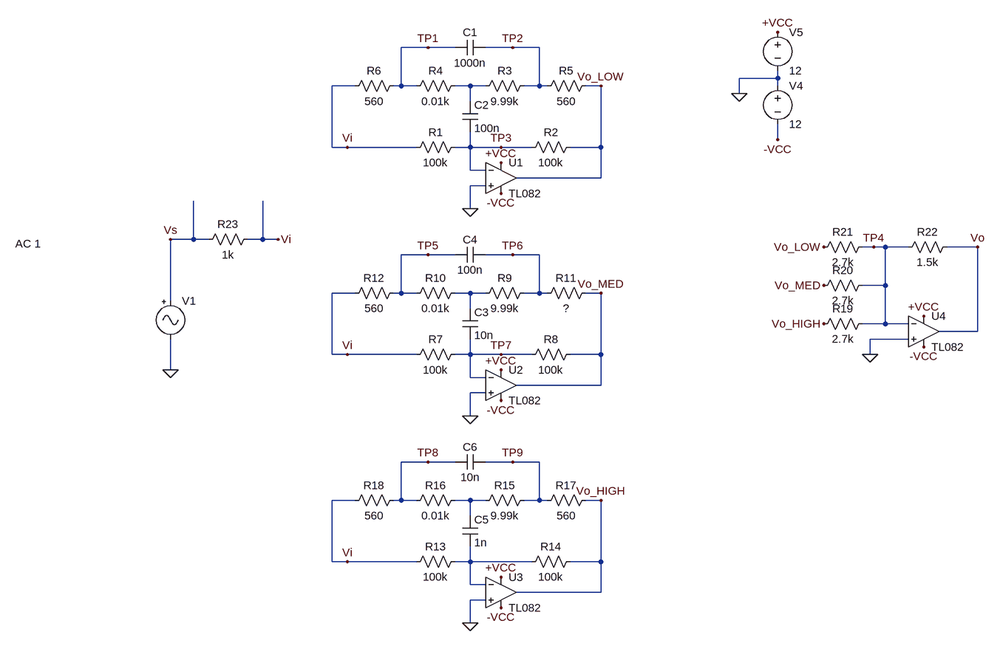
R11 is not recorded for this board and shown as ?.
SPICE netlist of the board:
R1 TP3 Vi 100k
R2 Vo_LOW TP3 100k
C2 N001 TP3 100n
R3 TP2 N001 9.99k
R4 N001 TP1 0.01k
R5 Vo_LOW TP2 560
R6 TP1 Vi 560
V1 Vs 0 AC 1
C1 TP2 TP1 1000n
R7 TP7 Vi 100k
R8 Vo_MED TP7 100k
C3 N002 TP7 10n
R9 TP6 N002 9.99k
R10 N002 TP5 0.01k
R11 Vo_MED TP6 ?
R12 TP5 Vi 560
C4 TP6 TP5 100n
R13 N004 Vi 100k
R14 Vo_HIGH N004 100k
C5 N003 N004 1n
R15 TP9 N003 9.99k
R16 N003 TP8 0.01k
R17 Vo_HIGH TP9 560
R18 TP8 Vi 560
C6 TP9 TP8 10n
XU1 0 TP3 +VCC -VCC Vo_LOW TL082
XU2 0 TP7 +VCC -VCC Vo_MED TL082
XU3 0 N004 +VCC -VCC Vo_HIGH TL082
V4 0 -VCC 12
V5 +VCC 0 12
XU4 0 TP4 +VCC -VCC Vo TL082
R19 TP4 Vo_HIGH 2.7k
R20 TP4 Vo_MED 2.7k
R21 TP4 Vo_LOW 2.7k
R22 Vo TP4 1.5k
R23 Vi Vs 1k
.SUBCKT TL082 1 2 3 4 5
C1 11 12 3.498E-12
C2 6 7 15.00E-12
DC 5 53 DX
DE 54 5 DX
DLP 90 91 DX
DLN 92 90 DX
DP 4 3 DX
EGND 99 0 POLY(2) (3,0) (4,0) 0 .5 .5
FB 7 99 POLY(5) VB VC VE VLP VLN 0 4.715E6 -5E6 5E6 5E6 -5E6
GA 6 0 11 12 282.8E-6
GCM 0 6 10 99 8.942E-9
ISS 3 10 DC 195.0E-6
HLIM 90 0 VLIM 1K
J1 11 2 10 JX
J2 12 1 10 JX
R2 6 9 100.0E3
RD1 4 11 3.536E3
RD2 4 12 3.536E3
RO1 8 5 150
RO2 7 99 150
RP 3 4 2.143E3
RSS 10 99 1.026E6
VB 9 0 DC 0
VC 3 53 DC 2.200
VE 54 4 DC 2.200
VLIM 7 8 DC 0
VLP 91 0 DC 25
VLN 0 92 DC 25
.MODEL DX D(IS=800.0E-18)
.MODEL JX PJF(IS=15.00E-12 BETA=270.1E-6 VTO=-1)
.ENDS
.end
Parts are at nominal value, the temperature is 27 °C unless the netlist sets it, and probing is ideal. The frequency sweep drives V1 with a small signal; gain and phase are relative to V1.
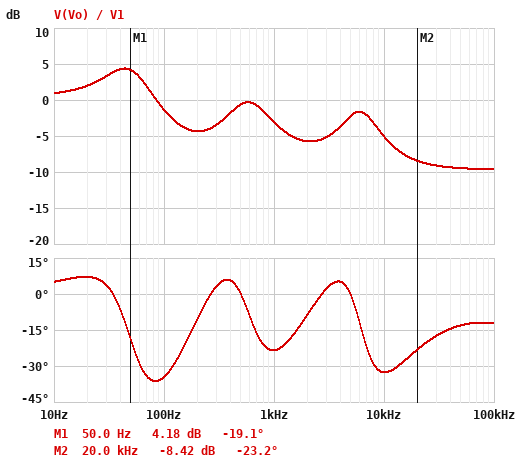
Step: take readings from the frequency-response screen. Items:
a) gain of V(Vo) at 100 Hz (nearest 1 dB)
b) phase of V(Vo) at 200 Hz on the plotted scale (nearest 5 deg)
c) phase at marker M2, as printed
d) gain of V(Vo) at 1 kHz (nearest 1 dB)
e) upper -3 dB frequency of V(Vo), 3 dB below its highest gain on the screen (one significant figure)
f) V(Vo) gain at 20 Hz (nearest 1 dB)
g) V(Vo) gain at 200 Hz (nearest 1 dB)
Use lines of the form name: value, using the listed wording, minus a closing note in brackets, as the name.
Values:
gain of V(Vo) at 100 Hz: -1 dB
phase of V(Vo) at 200 Hz on the plotted scale: -10 deg
phase at marker M2, as printed: -23.2 deg
gain of V(Vo) at 1 kHz: -3 dB
upper -3 dB frequency of V(Vo), 3 dB below its highest gain on the screen: 70 Hz
V(Vo) gain at 20 Hz: 2 dB
V(Vo) gain at 200 Hz: -4 dB
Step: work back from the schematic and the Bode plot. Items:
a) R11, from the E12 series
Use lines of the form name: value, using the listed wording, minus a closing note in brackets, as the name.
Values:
R11, from the E12 series: 1 kΩ
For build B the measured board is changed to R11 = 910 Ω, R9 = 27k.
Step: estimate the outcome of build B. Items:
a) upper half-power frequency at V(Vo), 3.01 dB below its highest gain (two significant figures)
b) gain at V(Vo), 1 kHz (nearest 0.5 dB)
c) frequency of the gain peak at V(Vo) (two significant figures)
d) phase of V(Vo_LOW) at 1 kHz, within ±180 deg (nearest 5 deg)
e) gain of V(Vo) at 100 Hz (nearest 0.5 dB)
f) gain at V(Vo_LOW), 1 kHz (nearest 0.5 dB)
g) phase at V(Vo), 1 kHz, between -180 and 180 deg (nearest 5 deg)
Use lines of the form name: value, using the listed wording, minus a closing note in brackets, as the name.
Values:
upper half-power frequency at V(Vo), 3.01 dB below its highest gain: 72 Hz
gain at V(Vo), 1 kHz: -3.5 dB
frequency of the gain peak at V(Vo): 43 Hz
phase of V(Vo_LOW) at 1 kHz, within ±180 deg: 155 deg
gain of V(Vo) at 100 Hz: -1.0 dB
gain at V(Vo_LOW), 1 kHz: -14.5 dB
phase at V(Vo), 1 kHz, between -180 and 180 deg: -30 deg
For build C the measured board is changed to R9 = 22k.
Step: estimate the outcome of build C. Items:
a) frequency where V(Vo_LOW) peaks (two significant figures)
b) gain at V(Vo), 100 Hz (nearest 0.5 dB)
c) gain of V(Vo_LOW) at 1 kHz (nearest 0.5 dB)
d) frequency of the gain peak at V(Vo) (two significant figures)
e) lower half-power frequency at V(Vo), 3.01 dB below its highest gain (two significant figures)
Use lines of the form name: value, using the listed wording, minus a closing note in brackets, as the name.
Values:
frequency where V(Vo_LOW) peaks: 48 Hz
gain at V(Vo), 100 Hz: -1.0 dB
gain of V(Vo_LOW) at 1 kHz: -14.5 dB
frequency of the gain peak at V(Vo): 43 Hz
lower half-power frequency at V(Vo), 3.01 dB below its highest gain: 13 Hz
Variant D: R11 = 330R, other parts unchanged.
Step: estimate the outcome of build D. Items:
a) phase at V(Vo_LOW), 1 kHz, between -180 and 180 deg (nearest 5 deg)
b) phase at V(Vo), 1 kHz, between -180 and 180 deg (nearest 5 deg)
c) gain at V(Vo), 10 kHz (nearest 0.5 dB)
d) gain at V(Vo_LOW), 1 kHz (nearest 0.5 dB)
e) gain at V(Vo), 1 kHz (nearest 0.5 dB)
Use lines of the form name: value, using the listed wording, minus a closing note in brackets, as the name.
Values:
phase at V(Vo_LOW), 1 kHz, between -180 and 180 deg: 155 deg
phase at V(Vo), 1 kHz, between -180 and 180 deg: -40 deg
gain at V(Vo), 10 kHz: -6.5 dB
gain at V(Vo_LOW), 1 kHz: -15.0 dB
gain at V(Vo), 1 kHz: -4.5 dB
